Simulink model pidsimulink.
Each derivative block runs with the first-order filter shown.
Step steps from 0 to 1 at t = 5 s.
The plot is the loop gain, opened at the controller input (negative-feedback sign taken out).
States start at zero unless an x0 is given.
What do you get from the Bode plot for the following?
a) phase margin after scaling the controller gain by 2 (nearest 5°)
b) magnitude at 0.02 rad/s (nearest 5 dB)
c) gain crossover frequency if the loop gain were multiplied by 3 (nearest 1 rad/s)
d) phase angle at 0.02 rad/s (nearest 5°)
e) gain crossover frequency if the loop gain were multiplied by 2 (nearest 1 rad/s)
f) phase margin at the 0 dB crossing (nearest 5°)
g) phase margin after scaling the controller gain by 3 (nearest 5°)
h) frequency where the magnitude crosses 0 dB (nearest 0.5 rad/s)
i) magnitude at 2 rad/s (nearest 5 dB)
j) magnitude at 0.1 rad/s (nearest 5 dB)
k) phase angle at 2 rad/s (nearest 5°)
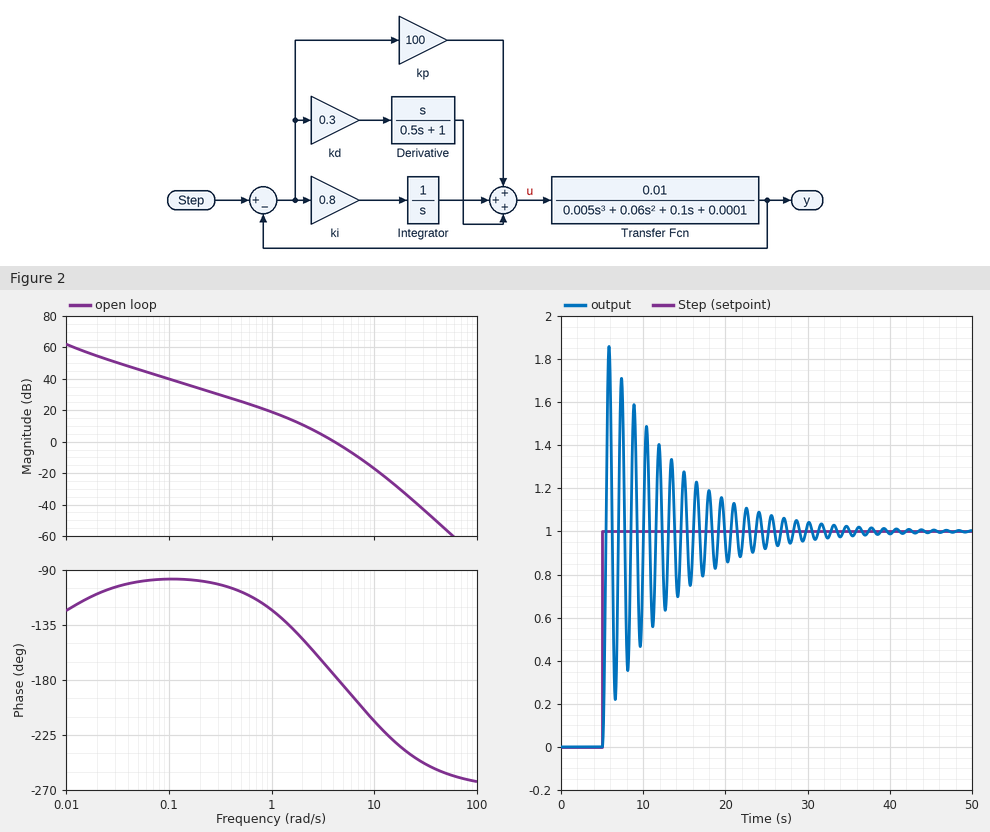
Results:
-10°
55 dB
7 rad/s
-110°
6 rad/s
5°
-20°
4.0 rad/s
10 dB
40 dB
-145°
